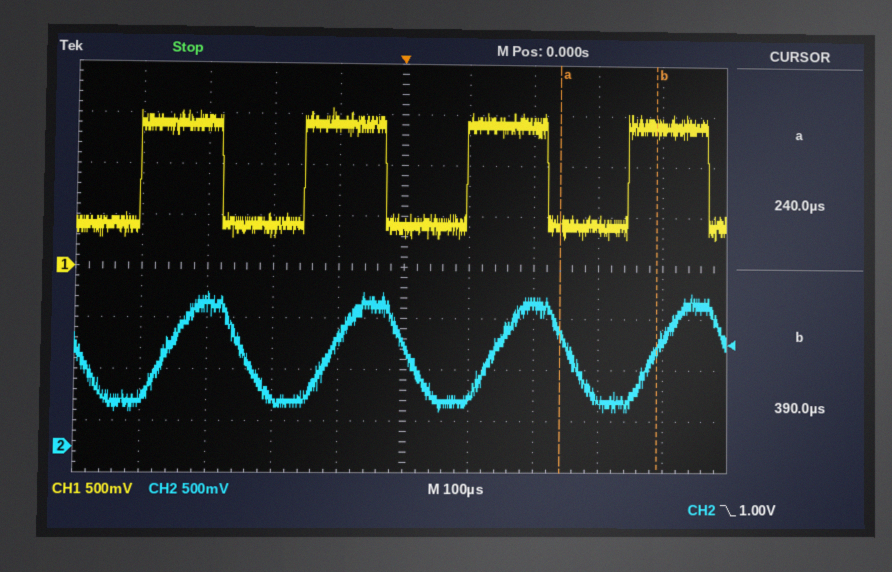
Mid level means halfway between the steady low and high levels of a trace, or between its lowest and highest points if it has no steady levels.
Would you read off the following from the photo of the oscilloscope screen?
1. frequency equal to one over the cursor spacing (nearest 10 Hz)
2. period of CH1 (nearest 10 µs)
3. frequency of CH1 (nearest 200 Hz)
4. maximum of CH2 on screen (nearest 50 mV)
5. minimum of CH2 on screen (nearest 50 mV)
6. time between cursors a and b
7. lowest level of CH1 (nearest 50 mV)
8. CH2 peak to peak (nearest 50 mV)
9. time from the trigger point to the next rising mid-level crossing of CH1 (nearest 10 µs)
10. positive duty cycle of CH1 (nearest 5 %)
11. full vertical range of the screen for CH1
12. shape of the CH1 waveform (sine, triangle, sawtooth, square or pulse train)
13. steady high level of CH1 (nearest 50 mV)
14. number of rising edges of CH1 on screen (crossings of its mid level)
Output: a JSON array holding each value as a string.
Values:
["6.67 kHz", "250 µs", "4.0 kHz", "1.50 V", "350 mV", "150 µs", "300 mV", "1.15 V", "100 µs", "50 %", "4 V", "square", "1.40 V", "4"]
